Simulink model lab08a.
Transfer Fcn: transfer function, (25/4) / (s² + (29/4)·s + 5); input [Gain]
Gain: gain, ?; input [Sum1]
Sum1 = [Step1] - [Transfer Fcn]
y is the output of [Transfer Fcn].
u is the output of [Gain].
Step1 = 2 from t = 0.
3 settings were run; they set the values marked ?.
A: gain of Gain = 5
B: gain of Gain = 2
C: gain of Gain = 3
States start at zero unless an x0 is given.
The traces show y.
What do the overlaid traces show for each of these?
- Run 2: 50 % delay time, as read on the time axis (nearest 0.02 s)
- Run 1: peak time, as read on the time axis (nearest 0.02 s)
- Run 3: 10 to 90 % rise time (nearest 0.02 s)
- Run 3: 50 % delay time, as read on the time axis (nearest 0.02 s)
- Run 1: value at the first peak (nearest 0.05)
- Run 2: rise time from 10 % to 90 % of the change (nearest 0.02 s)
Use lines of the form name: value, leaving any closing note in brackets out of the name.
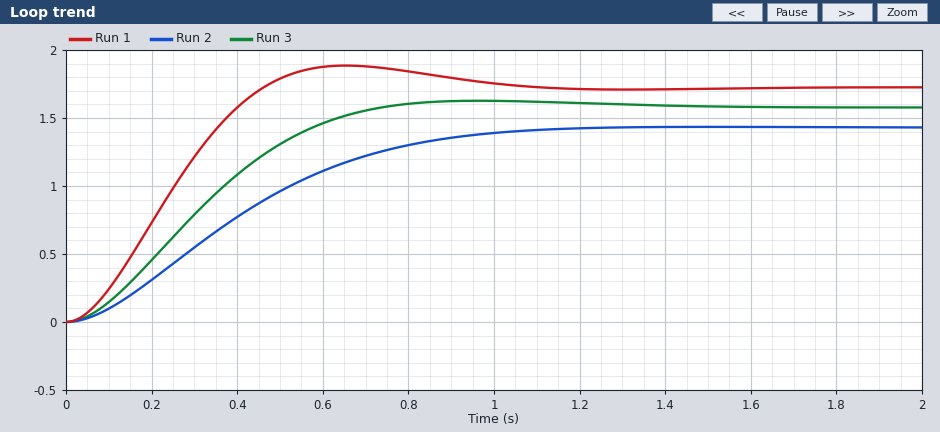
Run 2: 50 % delay time, as read on the time axis: 0.38 s
Run 1: peak time, as read on the time axis: 0.66 s
Run 3: 10 to 90 % rise time: 0.46 s
Run 3: 50 % delay time, as read on the time axis: 0.30 s
Run 1: value at the first peak: 1.90
Run 2: rise time from 10 % to 90 % of the change: 0.66 s
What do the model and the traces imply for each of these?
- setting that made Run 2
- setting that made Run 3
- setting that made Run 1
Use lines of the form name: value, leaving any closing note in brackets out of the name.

setting that made Run 2: B
setting that made Run 3: C
setting that made Run 1: A
